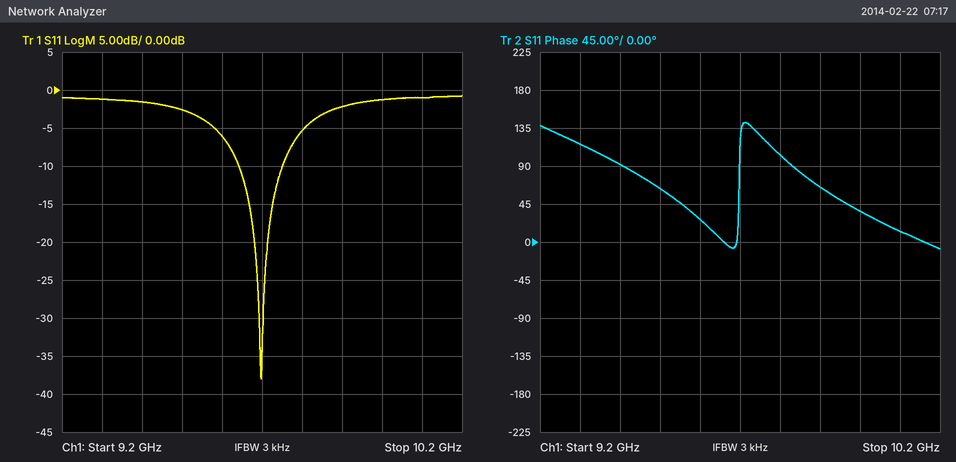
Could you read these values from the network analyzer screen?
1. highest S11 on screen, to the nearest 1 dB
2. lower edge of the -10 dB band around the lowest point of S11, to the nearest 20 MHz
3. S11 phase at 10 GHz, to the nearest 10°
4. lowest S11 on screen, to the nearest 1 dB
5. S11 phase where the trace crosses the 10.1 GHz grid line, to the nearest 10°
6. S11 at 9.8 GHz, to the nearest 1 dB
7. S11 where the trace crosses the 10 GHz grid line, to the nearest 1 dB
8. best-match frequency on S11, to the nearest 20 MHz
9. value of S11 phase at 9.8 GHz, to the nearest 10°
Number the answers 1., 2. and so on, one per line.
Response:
1. -1 dB
2. 9.64 GHz
3. 40°
4. -38 dB
5. 10°
6. -5 dB
7. -1 dB
8. 9.70 GHz
9. 100°
